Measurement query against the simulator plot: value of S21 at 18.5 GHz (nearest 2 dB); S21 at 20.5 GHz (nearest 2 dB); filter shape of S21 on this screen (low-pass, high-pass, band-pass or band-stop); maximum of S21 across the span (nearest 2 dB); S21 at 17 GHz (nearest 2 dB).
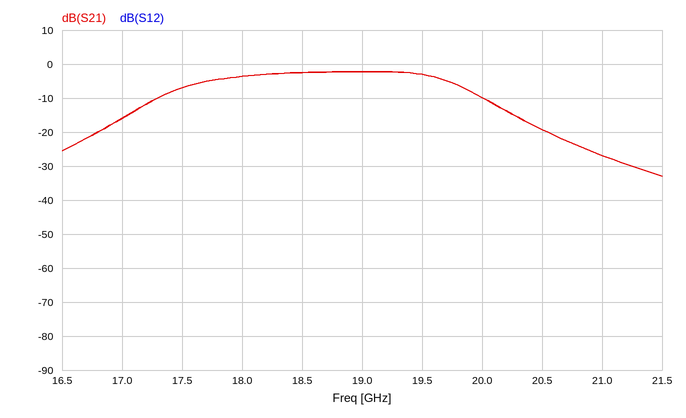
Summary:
-2 dB
-20 dB
band-pass
-2 dB
-16 dB
